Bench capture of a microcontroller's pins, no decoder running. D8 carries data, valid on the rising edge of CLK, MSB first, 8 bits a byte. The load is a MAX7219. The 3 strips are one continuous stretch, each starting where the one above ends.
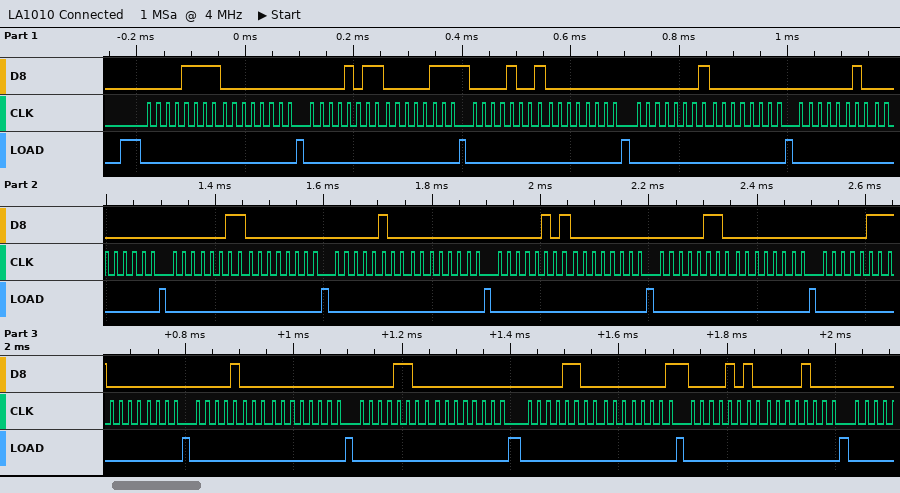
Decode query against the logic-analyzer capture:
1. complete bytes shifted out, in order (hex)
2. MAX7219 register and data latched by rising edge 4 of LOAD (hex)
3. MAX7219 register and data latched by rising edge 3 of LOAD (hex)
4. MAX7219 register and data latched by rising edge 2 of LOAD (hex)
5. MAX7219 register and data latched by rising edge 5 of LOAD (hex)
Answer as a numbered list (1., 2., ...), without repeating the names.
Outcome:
1. 0x0F 0x00 0x0B 0x07 0x09 0x00 0x01 0x00 0x02 0x00 0x03 0x00 0x04 0x00 0x05 0x00 0x06 0x00 0x07 0x00 0x08 0x00 0x0C 0x00 0x0C 0x01 0x0A 0x08
2. register 0x9, data 0x00
3. register 0xB, data 0x07
4. register 0xF, data 0x00
5. register 0x1, data 0x00
